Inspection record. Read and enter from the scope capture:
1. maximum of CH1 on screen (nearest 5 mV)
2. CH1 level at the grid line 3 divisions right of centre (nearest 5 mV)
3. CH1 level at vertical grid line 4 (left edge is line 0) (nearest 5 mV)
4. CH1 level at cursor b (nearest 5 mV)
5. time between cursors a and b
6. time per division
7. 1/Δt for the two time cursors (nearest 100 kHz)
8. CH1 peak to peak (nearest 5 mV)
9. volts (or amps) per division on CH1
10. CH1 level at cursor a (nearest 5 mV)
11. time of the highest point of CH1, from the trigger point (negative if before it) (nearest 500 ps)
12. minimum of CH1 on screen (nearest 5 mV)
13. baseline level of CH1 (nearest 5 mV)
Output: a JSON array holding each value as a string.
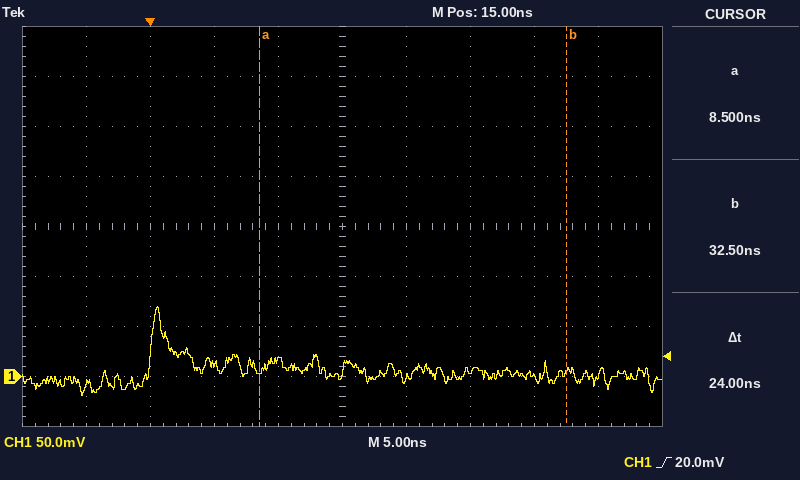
["70 mV", "0 mV", "15 mV", "5 mV", "24 ns", "5 ns", "41.7 MHz", "90 mV", "50 mV", "5 mV", "+500 ps", "-20 mV", "5 mV"]
